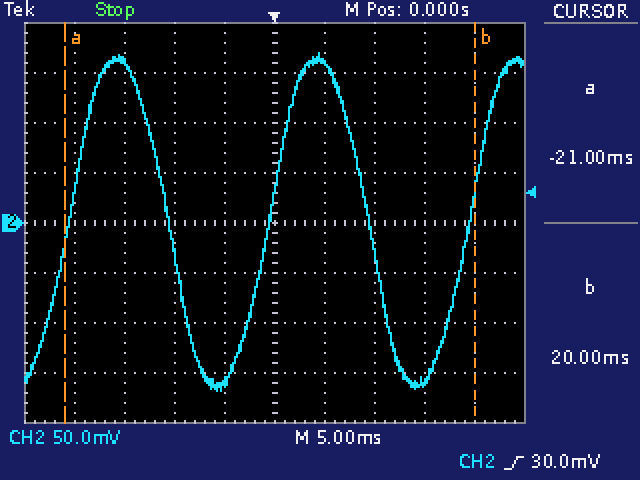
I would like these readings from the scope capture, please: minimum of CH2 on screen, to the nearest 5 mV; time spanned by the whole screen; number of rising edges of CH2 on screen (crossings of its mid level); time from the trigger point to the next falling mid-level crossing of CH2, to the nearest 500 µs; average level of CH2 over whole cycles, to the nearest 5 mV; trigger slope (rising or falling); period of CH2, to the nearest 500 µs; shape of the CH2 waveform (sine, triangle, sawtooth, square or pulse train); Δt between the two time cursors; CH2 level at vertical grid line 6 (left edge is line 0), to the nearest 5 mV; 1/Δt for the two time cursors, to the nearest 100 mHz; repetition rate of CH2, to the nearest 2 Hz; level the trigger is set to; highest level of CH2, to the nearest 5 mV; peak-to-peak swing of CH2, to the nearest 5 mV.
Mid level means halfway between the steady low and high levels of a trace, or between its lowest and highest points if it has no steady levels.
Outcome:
-170 mV
50 ms
3
9.5 ms
0 mV
rising
20.0 ms
sine
41.0 ms
160 mV
24.4 Hz
50 Hz
30.0 mV
170 mV
340 mV
